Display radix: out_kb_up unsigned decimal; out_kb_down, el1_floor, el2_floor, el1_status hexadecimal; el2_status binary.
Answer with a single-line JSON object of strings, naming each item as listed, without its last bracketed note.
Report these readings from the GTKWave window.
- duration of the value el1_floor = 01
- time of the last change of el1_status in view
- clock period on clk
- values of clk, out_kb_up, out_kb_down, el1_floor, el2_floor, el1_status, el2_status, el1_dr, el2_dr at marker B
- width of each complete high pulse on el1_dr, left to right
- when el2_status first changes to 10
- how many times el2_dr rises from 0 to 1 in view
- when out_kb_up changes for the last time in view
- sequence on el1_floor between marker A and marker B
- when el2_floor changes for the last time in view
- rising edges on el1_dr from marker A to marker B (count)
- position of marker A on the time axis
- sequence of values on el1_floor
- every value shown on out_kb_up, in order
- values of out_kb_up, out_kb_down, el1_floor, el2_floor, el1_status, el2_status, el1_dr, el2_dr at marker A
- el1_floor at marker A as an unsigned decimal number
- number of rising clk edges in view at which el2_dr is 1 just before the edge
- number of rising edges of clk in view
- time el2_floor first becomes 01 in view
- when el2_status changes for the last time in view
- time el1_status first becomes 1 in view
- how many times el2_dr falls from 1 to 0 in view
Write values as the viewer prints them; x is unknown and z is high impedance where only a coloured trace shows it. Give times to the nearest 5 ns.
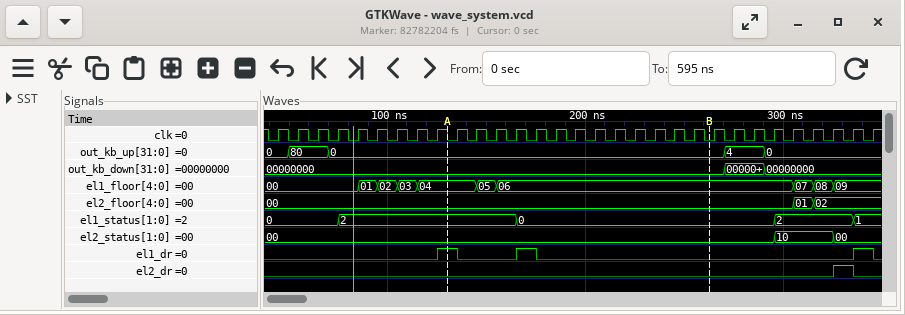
{"duration of the value el1_floor = 01": "10 ns", "time of the last change of el1_status in view": "335 ns", "clock period on clk": "10 ns", "values of clk, out_kb_up, out_kb_down, el1_floor, el2_floor, el1_status, el2_status, el1_dr, el2_dr at marker B": "clk=0, out_kb_up=0, out_kb_down=00000000, el1_floor=06, el2_floor=00, el1_status=0, el2_status=00, el1_dr=0, el2_dr=0", "width of each complete high pulse on el1_dr, left to right": "10 ns, 10 ns, 10 ns", "when el2_status first changes to 10": "295 ns", "how many times el2_dr rises from 0 to 1 in view": "1", "when out_kb_up changes for the last time in view": "290 ns", "sequence on el1_floor between marker A and marker B": "04, 05, 06", "when el2_floor changes for the last time in view": "315 ns", "rising edges on el1_dr from marker A to marker B": "1", "position of marker A on the time axis": "130 ns", "sequence of values on el1_floor": "00, 01, 02, 03, 04, 05, 06, 07, 08, 09", "every value shown on out_kb_up, in order": "0, 80, 0, 4, 0", "values of out_kb_up, out_kb_down, el1_floor, el2_floor, el1_status, el2_status, el1_dr, el2_dr at marker A": "out_kb_up=0, out_kb_down=00000000, el1_floor=04, el2_floor=00, el1_status=2, el2_status=00, el1_dr=1, el2_dr=0", "el1_floor at marker A as an unsigned decimal number": "4", "number of rising clk edges in view at which el2_dr is 1 just before the edge": "1", "number of rising edges of clk in view": "31", "time el2_floor first becomes 01 in view": "305 ns", "when el2_status changes for the last time in view": "325 ns", "time el1_status first becomes 1 in view": "335 ns", "how many times el2_dr falls from 1 to 0 in view": "1"}
